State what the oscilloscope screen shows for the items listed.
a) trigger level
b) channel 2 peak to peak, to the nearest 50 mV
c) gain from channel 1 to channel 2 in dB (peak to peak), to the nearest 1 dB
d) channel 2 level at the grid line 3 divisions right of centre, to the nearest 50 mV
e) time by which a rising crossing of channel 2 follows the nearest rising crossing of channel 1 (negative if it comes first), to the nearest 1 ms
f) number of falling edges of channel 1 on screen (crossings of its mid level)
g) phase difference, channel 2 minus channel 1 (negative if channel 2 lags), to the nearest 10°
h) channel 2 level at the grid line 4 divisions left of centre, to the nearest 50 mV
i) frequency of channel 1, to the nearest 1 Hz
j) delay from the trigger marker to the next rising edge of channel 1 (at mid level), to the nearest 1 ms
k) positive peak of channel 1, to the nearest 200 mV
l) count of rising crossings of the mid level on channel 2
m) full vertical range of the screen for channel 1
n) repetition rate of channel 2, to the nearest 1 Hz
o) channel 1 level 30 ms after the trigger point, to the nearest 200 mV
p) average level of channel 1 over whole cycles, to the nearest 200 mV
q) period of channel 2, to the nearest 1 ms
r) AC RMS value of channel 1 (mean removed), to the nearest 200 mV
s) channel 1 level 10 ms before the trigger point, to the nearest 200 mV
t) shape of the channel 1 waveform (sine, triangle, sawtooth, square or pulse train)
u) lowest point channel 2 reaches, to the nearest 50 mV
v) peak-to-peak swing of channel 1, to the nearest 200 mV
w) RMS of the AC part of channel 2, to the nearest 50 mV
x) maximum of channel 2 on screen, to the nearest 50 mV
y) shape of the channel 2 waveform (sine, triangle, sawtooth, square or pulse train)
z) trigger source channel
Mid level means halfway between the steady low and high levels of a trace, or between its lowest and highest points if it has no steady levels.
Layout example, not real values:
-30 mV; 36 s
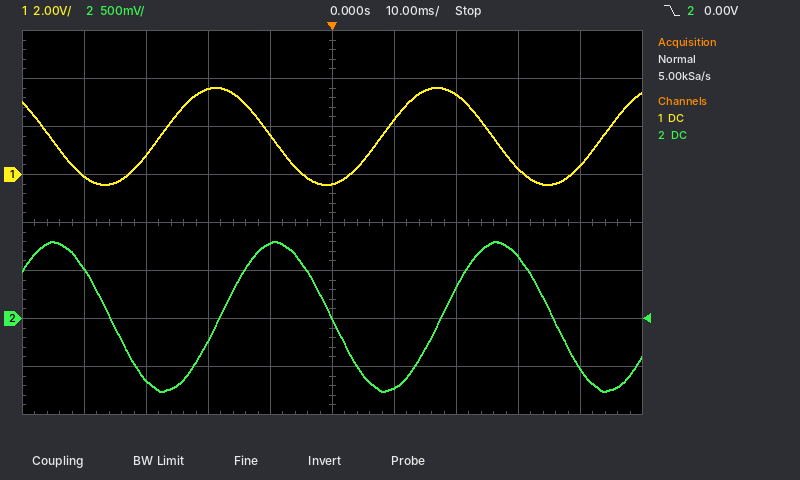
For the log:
0.00 V; 1.55 V; -8 dB; 650 mV; +10 ms; 3; -100°; 500 mV; 28 Hz; 8 ms; 3.6 V; 2; 16 V; 28 Hz; 200 mV; 1.6 V; 36 ms; 1.4 V; 1.6 V; sine; -750 mV; 4.0 V; 550 mV; 800 mV; sine; channel 2
